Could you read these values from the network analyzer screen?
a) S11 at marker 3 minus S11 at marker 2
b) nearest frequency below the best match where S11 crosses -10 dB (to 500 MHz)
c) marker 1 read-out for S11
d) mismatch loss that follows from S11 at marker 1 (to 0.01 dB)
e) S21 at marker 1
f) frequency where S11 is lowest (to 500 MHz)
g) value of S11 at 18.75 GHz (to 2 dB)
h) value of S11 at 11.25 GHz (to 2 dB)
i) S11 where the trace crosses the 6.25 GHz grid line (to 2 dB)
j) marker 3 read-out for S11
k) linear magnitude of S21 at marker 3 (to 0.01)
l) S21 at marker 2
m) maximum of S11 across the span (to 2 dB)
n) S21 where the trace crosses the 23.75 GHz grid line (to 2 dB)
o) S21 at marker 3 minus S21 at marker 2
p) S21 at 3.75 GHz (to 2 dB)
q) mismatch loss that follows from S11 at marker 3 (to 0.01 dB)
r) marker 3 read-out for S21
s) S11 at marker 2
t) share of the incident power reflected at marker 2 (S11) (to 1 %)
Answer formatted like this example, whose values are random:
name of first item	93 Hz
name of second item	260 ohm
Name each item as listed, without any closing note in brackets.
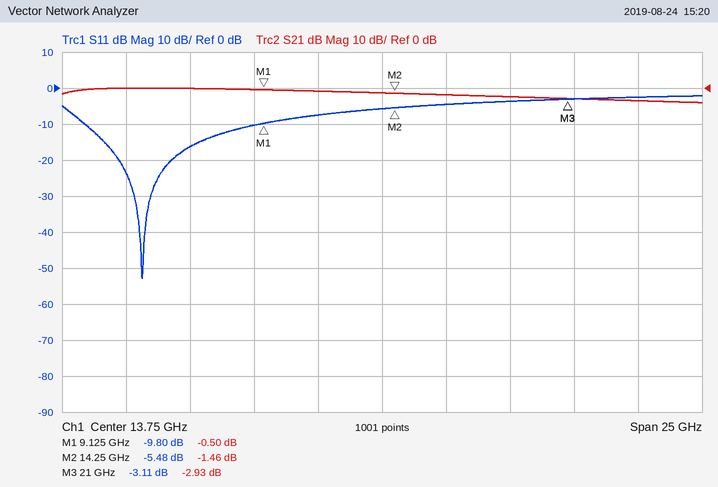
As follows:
S11 at marker 3 minus S11 at marker 2	2.37 dB
nearest frequency below the best match where S11 crosses -10 dB	2.0 GHz
marker 1 read-out for S11	-9.80 dB
mismatch loss that follows from S11 at marker 1	0.48 dB
S21 at marker 1	-0.50 dB
frequency where S11 is lowest	4.5 GHz
value of S11 at 18.75 GHz	-4 dB
value of S11 at 11.25 GHz	-8 dB
S11 where the trace crosses the 6.25 GHz grid line	-16 dB
marker 3 read-out for S11	-3.11 dB
linear magnitude of S21 at marker 3	0.71
S21 at marker 2	-1.46 dB
maximum of S11 across the span	-2 dB
S21 where the trace crosses the 23.75 GHz grid line	-4 dB
S21 at marker 3 minus S21 at marker 2	-1.47 dB
S21 at 3.75 GHz	0 dB
mismatch loss that follows from S11 at marker 3	2.91 dB
marker 3 read-out for S21	-2.93 dB
S11 at marker 2	-5.48 dB
share of the incident power reflected at marker 2 (S11)	28 %
